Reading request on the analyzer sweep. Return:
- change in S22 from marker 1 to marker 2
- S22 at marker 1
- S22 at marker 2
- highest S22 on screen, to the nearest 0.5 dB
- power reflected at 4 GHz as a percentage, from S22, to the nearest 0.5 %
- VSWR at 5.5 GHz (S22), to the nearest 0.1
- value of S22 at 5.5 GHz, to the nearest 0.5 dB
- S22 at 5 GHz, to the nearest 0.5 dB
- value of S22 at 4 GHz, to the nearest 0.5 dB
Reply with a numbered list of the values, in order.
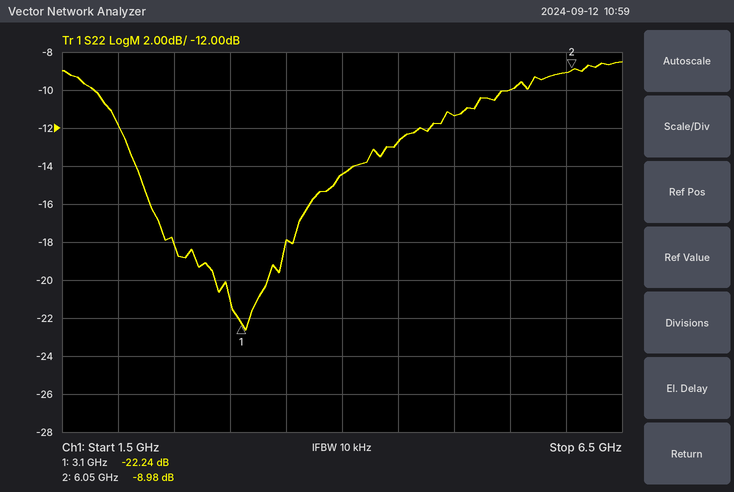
1. 13.26 dB
2. -22.24 dB
3. -8.98 dB
4. -8.5 dB
5. 3.5 %
6. 1.9
7. -10.0 dB
8. -11.5 dB
9. -14.5 dB
